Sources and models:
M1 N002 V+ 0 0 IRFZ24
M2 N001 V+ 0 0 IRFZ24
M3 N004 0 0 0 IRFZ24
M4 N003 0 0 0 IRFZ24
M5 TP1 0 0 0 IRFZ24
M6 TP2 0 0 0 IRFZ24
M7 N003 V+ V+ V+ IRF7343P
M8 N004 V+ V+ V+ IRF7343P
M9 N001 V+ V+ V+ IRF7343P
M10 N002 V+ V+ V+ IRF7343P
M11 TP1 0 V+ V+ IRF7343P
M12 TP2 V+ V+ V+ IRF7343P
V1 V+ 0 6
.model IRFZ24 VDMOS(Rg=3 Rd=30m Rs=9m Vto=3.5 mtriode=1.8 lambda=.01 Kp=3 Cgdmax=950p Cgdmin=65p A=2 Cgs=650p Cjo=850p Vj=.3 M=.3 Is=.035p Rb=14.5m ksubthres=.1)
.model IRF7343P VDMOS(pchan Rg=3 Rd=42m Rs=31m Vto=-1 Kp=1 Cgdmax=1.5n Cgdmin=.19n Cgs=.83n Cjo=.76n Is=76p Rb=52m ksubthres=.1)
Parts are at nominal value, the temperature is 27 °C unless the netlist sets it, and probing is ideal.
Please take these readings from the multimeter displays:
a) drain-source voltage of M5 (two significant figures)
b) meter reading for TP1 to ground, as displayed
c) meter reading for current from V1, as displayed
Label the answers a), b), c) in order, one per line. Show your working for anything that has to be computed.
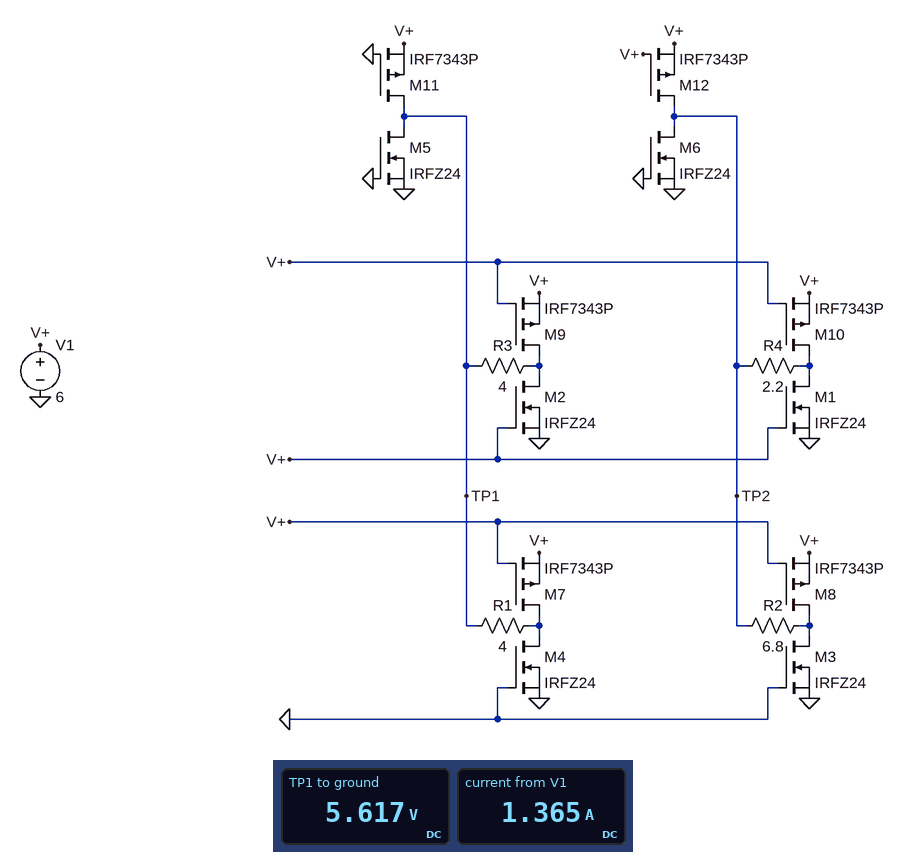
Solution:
a) 5.617 V = 5.6 V
b) 5.617 V
c) 1.365 A
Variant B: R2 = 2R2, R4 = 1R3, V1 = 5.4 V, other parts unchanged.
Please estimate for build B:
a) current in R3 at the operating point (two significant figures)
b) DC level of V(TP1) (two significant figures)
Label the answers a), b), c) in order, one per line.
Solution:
a) 1.2 A
b) 5.0 V
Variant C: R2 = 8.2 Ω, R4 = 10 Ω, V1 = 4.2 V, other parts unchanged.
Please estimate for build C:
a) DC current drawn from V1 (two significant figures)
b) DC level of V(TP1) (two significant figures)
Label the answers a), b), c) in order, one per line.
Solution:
a) 730 mA
b) 3.9 V
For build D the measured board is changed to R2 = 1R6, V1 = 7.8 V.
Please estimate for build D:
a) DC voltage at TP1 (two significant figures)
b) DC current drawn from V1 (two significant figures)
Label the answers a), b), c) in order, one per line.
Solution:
a) 7.4 V
b) 1.8 A
